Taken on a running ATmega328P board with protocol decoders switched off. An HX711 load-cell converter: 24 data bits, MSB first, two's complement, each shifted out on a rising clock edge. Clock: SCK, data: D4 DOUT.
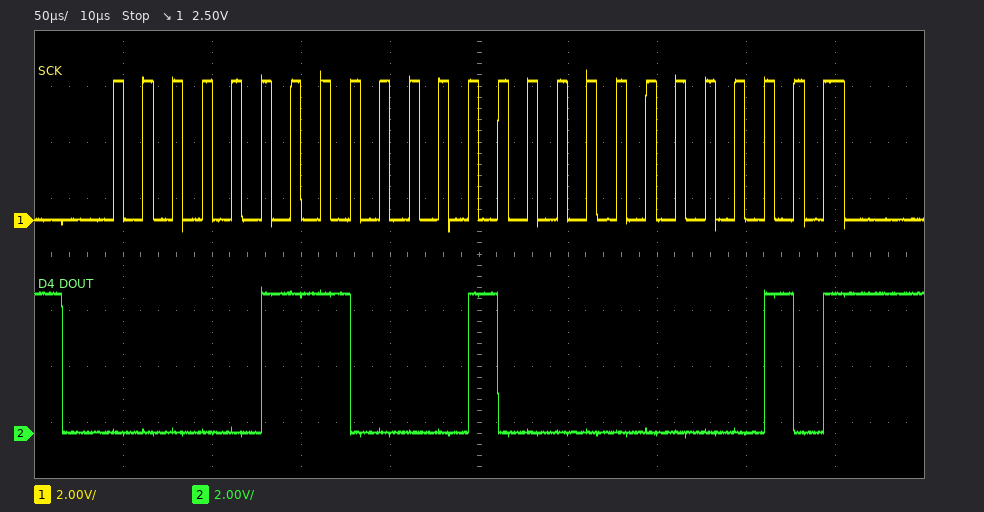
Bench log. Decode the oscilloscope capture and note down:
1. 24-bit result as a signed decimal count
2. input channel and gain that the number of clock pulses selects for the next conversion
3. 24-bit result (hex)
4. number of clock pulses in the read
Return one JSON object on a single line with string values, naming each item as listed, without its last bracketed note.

{"24-bit result as a signed decimal count": "460802", "input channel and gain that the number of clock pulses selects for the next conversion": "channel A, gain 128", "24-bit result": "0x070802", "number of clock pulses in the read": "25"}
